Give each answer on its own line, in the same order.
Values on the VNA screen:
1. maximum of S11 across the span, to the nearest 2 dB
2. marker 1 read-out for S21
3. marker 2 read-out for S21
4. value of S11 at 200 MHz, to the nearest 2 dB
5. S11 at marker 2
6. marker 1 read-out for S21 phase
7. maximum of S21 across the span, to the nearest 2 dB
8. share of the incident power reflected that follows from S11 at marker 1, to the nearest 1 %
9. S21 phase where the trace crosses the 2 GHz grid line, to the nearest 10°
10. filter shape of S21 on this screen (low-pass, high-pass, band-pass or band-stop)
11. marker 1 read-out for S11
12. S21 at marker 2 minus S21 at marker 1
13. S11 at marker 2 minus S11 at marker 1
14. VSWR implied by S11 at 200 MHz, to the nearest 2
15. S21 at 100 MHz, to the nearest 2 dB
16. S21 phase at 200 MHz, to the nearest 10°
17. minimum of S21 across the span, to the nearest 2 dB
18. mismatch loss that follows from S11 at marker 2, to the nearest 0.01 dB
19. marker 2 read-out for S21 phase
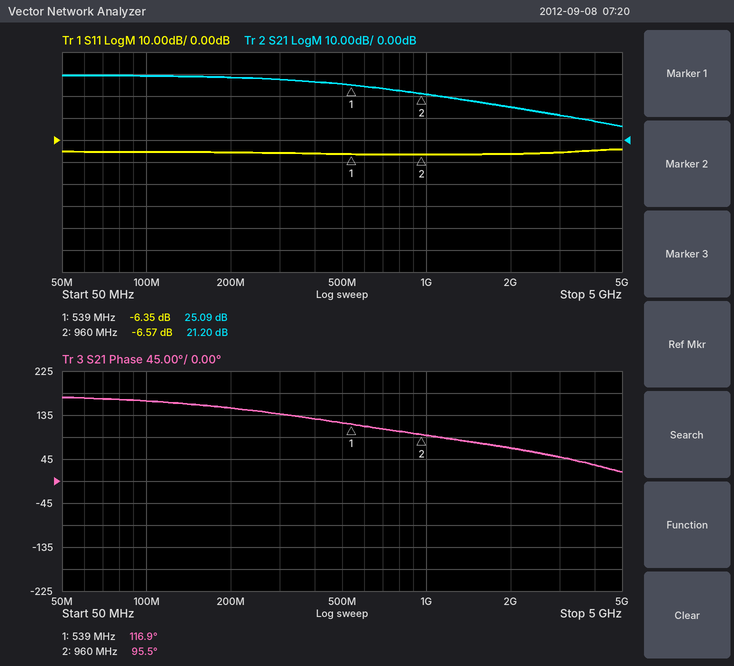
-4 dB
25.09 dB
21.20 dB
-6 dB
-6.57 dB
116.9°
30 dB
23 %
70°
low-pass
-6.35 dB
-3.89 dB
-0.22 dB
4
30 dB
150°
6 dB
1.08 dB
95.5°
